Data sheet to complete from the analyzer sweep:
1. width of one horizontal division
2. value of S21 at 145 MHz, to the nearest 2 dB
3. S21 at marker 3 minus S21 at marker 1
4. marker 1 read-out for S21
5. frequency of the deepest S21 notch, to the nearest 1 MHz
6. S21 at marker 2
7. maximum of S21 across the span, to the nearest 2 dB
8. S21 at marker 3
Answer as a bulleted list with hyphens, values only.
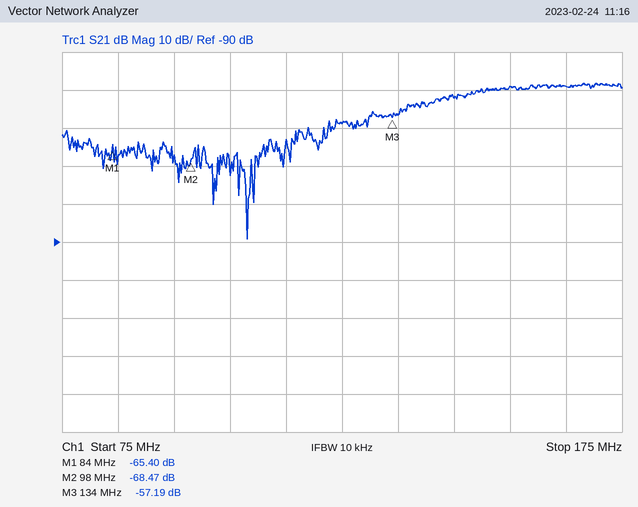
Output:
- 10 MHz
- -52 dB
- 8.21 dB
- -65.40 dB
- 108 MHz
- -68.47 dB
- -48 dB
- -57.19 dB
